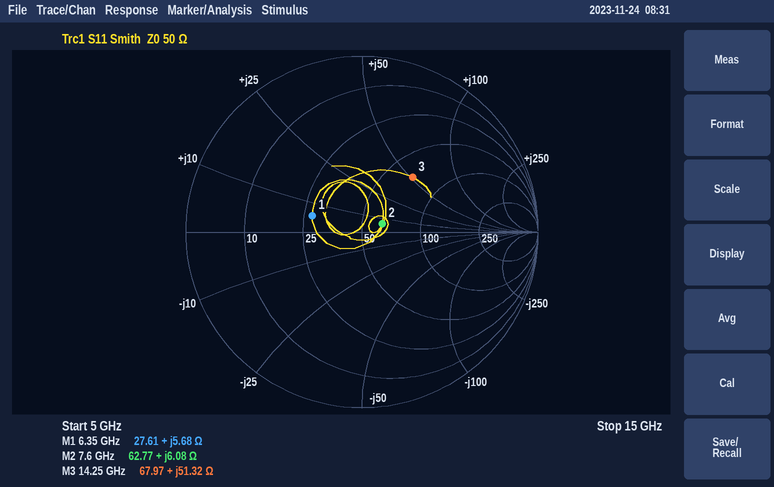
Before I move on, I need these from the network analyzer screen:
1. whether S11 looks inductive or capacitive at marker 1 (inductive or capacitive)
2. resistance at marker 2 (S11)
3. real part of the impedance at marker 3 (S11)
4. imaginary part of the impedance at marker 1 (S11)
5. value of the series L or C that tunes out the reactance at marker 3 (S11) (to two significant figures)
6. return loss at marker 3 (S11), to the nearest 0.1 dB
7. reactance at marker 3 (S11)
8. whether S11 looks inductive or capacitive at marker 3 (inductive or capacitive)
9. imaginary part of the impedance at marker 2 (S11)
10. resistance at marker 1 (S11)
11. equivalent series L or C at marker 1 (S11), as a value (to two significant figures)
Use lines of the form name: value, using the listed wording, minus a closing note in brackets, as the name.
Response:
whether S11 looks inductive or capacitive at marker 1: inductive
resistance at marker 2: 62.77 Ω
real part of the impedance at marker 3: 67.97 Ω
imaginary part of the impedance at marker 1: +5.68 Ω
value of the series L or C that tunes out the reactance at marker 3 (S11): 220 fF
return loss at marker 3 (S11), to the nearest 0.1 dB: 7.5 dB
reactance at marker 3: +51.32 Ω
whether S11 looks inductive or capacitive at marker 3: inductive
imaginary part of the impedance at marker 2: +6.08 Ω
resistance at marker 1: 27.61 Ω
equivalent series L or C at marker 1 (S11), as a value: 140 pH
